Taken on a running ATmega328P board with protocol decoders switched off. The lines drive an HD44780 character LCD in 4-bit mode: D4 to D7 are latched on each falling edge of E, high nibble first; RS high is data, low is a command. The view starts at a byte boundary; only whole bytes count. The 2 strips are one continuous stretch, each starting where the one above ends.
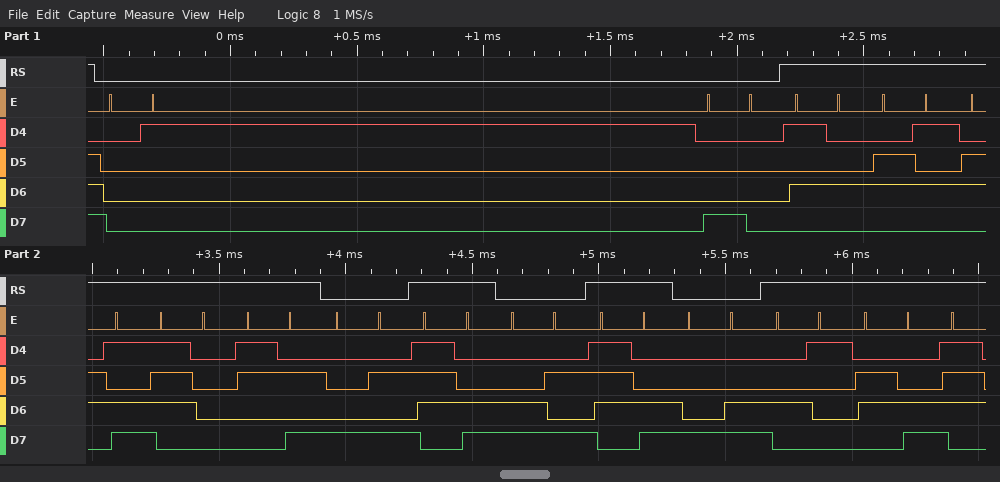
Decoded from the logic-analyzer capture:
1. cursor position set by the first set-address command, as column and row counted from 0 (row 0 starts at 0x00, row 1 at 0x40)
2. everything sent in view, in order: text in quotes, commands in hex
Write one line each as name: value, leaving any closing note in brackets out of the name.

cursor position set by the first set-address command, as column and row counted from 0: column 0, row 0
everything sent in view, in order: text in quotes, commands in hex: 0x01 0x80 "Temp:" 0x8A "|" 0xCA "|" 0x8C "Al"
